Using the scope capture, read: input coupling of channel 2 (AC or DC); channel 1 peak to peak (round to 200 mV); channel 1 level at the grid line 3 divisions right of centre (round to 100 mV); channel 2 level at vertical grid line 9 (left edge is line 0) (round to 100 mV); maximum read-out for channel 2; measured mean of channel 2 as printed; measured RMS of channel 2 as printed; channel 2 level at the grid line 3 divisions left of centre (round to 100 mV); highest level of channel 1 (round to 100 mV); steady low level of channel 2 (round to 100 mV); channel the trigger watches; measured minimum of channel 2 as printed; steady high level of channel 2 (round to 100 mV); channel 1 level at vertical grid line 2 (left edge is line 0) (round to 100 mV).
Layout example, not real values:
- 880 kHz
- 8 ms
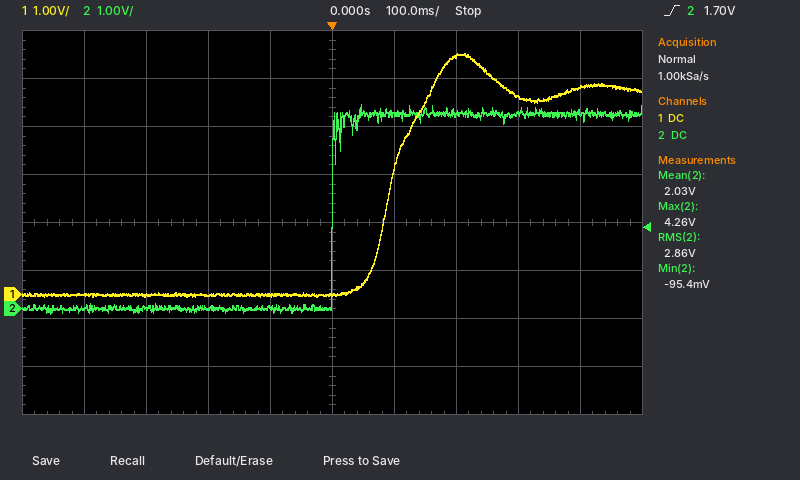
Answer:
- DC
- 5.0 V
- 4.1 V
- 4.1 V
- 4.26 V
- 2.03 V
- 2.86 V
- 0.0 V
- 5.0 V
- 0.0 V
- channel 2
- -95.4 mV
- 4.1 V
- 0.0 V
